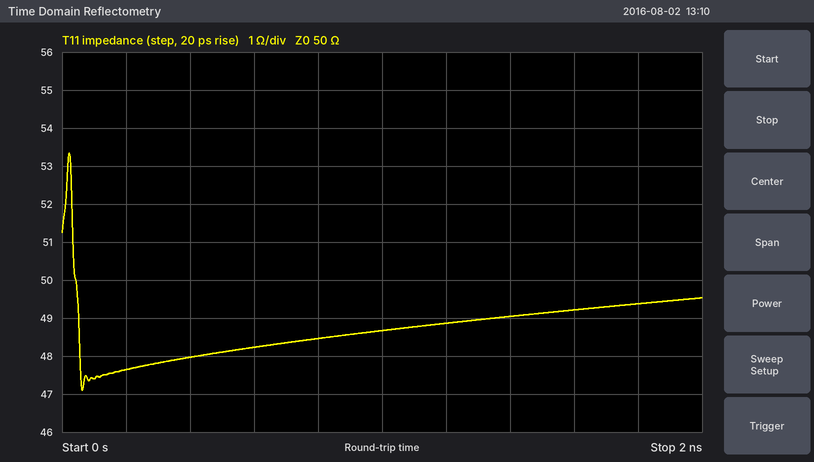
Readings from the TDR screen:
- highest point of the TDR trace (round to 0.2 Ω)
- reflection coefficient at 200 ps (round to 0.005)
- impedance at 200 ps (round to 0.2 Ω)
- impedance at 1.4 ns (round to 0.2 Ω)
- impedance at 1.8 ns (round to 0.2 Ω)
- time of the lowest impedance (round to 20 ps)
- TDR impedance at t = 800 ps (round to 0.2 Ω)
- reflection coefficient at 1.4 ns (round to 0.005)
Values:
53.4 Ω
-0.025
47.6 Ω
49.0 Ω
49.4 Ω
60 ps
48.4 Ω
-0.010
